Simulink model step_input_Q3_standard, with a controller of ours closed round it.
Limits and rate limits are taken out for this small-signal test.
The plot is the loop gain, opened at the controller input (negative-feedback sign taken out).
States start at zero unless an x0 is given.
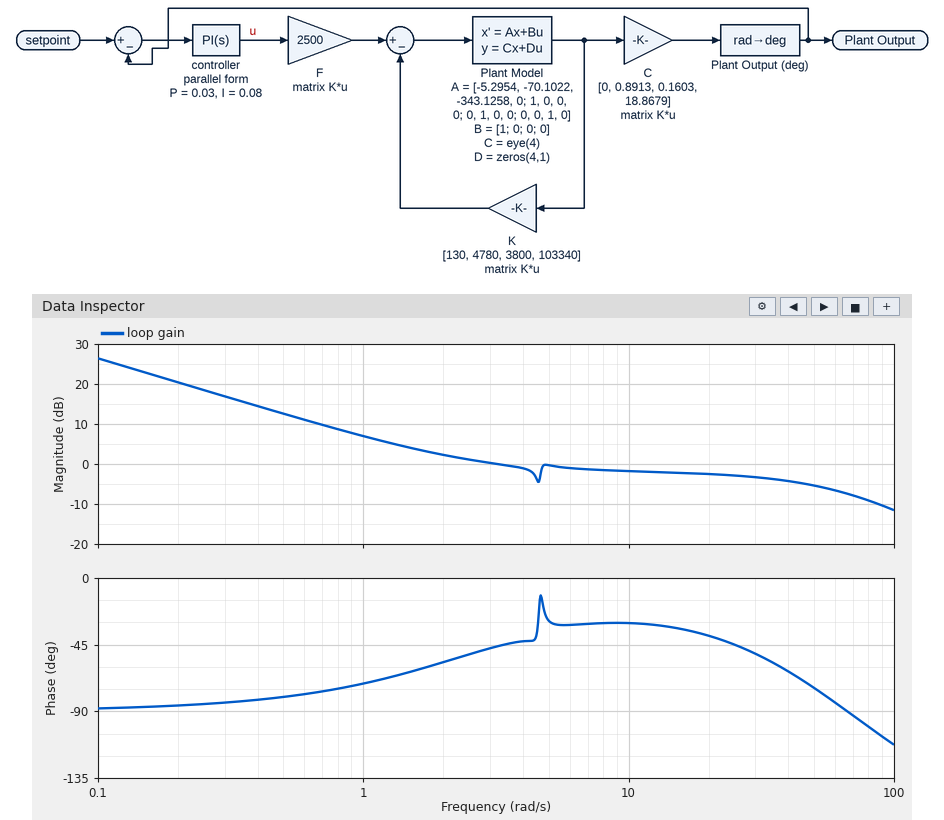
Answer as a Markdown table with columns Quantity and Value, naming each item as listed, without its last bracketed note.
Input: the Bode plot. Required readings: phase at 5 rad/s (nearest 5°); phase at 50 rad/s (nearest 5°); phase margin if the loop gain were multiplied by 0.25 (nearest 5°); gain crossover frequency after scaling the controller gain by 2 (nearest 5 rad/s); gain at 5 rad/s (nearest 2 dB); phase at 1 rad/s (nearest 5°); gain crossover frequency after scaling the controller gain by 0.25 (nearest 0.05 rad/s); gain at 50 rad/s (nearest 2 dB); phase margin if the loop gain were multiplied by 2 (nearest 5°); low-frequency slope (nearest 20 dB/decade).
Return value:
| Quantity | Value |
|---|---|
| phase at 5 rad/s | -30° |
| phase at 50 rad/s | -75° |
| phase margin if the loop gain were multiplied by 0.25 | 100° |
| gain crossover frequency after scaling the controller gain by 2 | 55 rad/s |
| gain at 5 rad/s | 0 dB |
| phase at 1 rad/s | -70° |
| gain crossover frequency after scaling the controller gain by 0.25 | 0.55 rad/s |
| gain at 50 rad/s | -6 dB |
| phase margin if the loop gain were multiplied by 2 | 100° |
| low-frequency slope | -20 dB/decade |
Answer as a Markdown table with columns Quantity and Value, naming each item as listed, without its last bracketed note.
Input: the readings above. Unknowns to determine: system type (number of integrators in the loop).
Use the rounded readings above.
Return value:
| Quantity | Value |
|---|---|
| system type | 1 |
